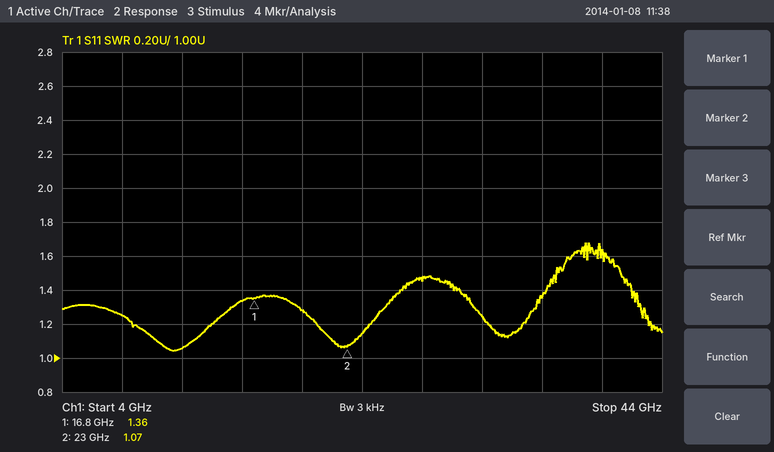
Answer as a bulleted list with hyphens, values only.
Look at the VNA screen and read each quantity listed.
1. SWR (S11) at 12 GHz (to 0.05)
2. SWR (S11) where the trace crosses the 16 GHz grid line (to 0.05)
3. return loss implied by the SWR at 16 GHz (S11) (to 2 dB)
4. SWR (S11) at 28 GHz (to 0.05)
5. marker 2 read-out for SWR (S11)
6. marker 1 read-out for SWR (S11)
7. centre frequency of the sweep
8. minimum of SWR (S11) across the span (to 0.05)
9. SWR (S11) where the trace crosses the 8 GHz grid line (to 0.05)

- 1.05
- 1.35
- 16 dB
- 1.45
- 1.07
- 1.36
- 24 GHz
- 1.05
- 1.25
